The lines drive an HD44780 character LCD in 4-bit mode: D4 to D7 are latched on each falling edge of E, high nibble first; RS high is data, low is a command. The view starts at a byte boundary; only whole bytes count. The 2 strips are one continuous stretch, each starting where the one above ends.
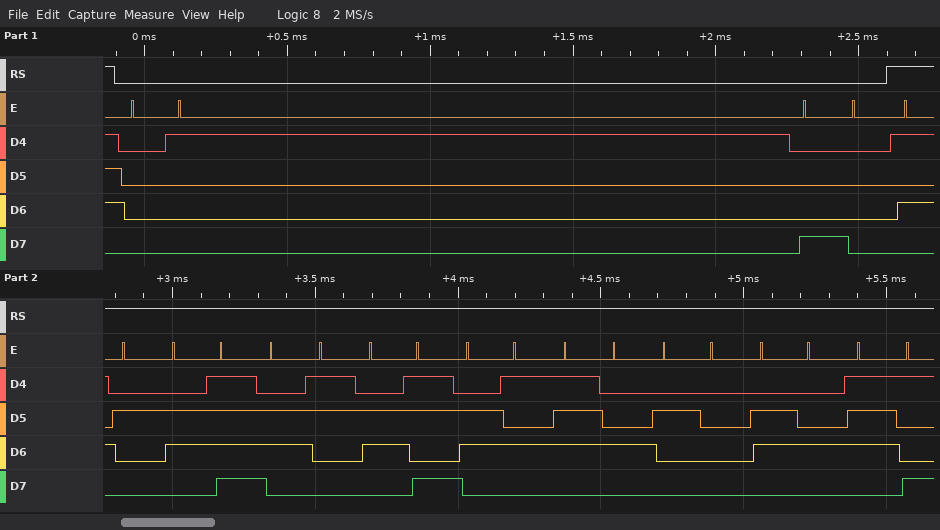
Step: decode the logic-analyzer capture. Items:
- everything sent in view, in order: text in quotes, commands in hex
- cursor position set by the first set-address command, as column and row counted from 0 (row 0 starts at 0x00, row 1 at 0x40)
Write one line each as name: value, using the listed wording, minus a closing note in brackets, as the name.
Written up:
everything sent in view, in order: text in quotes, commands in hex: 0x01 0x80 "Rocket dy"
cursor position set by the first set-address command, as column and row counted from 0: column 0, row 0
